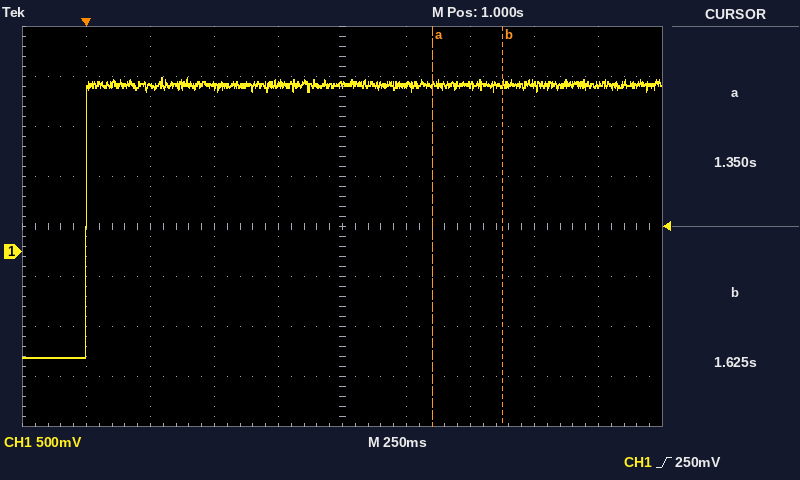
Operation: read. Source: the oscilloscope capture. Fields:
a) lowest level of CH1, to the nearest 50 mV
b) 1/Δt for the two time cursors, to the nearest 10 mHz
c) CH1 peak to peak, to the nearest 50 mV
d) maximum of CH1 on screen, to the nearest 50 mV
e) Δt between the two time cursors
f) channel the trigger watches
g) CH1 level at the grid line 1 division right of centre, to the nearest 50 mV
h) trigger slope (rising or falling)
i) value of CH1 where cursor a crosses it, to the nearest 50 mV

-1.05 V
3.64 Hz
2.80 V
1.75 V
275 ms
CH1
1.65 V
rising
1.65 V
